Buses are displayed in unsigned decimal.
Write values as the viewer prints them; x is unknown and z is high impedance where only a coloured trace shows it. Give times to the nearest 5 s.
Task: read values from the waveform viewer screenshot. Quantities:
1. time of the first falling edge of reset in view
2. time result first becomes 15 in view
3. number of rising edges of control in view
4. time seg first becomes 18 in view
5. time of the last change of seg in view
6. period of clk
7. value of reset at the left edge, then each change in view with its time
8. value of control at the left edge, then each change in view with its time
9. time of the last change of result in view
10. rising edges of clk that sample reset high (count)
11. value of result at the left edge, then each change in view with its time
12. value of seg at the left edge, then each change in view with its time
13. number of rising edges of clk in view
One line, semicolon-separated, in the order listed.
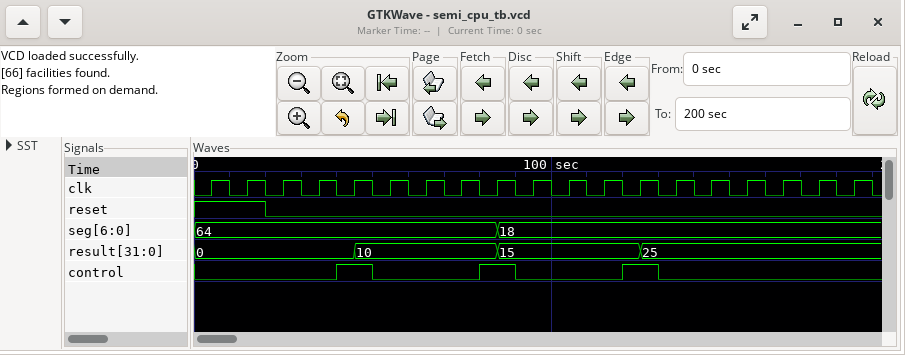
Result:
20 s; 85 s; 3; 85 s; 85 s; 10 s; 1, 0 at 20 s; 0, 1 at 40 s, 0 at 50 s, 1 at 80 s, 0 at 90 s, 1 at 120 s, 0 at 130 s; 125 s; 2; 0, 10 at 45 s, 15 at 85 s, 25 at 125 s; 64, 18 at 85 s; 19
